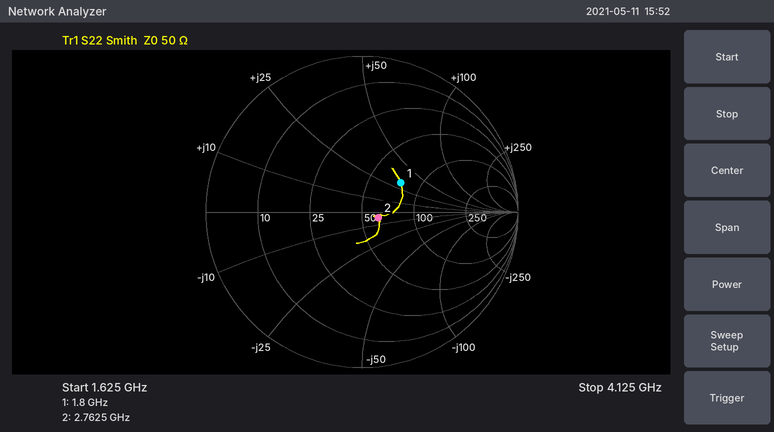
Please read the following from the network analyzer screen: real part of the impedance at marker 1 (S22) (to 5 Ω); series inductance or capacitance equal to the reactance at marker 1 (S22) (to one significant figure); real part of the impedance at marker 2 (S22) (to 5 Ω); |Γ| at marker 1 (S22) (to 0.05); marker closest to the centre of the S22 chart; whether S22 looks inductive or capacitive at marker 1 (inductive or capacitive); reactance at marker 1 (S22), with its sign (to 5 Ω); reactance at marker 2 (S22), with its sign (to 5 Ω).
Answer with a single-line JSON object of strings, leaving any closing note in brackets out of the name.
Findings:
{"real part of the impedance at marker 1 (S22)": "75 Ω", "series inductance or capacitance equal to the reactance at marker 1 (S22)": "3 nH", "real part of the impedance at marker 2 (S22)": "60 Ω", "|Γ| at marker 1 (S22)": "0.30", "marker closest to the centre of the S22 chart": "marker 2", "whether S22 looks inductive or capacitive at marker 1": "inductive", "reactance at marker 1 (S22), with its sign": "+30 Ω", "reactance at marker 2 (S22), with its sign": "-5 Ω"}
